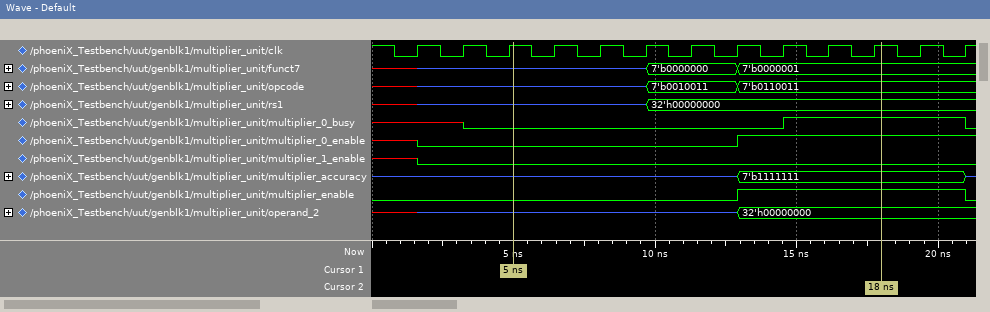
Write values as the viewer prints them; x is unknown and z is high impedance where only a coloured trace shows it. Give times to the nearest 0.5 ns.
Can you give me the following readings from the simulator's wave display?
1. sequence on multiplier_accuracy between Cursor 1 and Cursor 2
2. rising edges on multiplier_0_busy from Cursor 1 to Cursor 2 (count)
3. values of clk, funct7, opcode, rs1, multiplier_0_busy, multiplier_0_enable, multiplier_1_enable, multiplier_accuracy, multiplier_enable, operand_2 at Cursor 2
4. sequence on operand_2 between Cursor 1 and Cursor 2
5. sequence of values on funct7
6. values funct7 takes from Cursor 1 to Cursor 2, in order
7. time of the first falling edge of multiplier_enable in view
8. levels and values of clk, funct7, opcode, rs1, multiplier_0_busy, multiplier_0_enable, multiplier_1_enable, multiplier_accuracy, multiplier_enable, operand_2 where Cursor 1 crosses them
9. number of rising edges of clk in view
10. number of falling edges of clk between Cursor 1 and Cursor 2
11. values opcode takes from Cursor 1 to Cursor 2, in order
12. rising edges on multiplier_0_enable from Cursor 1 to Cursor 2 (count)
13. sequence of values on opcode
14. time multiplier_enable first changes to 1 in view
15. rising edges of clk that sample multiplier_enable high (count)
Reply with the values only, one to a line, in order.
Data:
z, 7'b1111111
1
clk=1, funct7=7'b0000001, opcode=7'b0110011, rs1=32'h00000000, multiplier_0_busy=1, multiplier_0_enable=1, multiplier_1_enable=0, multiplier_accuracy=7'b1111111, multiplier_enable=1, operand_2=32'h00000000
z, 32'h00000000
x, z, 7'b0000000, 7'b0000001
z, 7'b0000000, 7'b0000001
21 ns
clk=1, funct7=z, opcode=z, rs1=z, multiplier_0_busy=0, multiplier_0_enable=0, multiplier_1_enable=0, multiplier_accuracy=z, multiplier_enable=0, operand_2=z
13
8
z, 7'b0010011, 7'b0110011
1
x, z, 7'b0010011, 7'b0110011
13 ns
5
